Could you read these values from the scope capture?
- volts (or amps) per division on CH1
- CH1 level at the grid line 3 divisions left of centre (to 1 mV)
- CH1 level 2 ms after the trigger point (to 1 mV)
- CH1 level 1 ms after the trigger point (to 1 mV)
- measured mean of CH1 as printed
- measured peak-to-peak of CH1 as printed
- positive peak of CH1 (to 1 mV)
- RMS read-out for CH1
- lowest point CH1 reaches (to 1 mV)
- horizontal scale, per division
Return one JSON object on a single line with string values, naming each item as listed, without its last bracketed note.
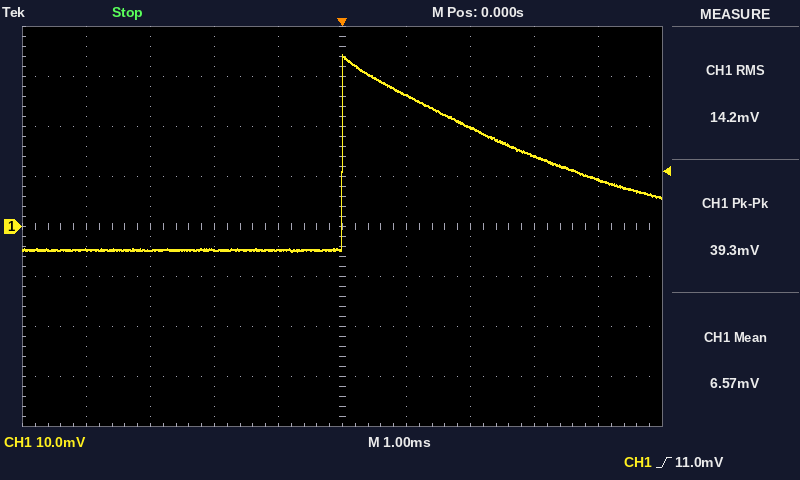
{"volts (or amps) per division on CH1": "10 mV", "CH1 level at the grid line 3 divisions left of centre": "-5 mV", "CH1 level 2 ms after the trigger point": "20 mV", "CH1 level 1 ms after the trigger point": "26 mV", "measured mean of CH1 as printed": "6.57 mV", "measured peak-to-peak of CH1 as printed": "39.3 mV", "positive peak of CH1": "34 mV", "RMS read-out for CH1": "14.2 mV", "lowest point CH1 reaches": "-5 mV", "horizontal scale, per division": "1 ms"}
